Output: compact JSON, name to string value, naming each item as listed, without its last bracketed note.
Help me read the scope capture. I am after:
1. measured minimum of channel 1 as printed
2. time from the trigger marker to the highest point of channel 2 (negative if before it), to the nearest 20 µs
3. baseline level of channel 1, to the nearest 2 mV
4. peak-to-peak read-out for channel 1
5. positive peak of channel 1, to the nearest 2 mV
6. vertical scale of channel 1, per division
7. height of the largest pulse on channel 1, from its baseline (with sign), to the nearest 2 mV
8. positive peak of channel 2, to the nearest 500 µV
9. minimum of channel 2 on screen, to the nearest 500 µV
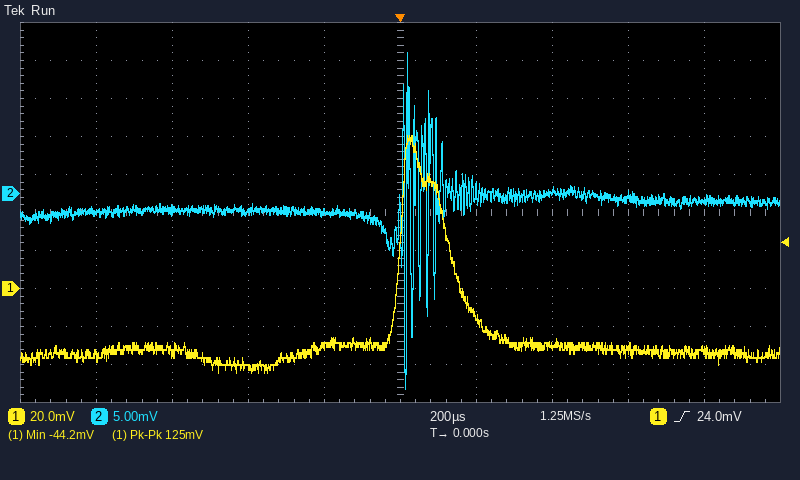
{"measured minimum of channel 1 as printed": "-44.2 mV", "time from the trigger marker to the highest point of channel 2 (negative if before it), to the nearest 20 µs": "+20 µs", "baseline level of channel 1, to the nearest 2 mV": "-32 mV", "peak-to-peak read-out for channel 1": "125 mV", "positive peak of channel 1, to the nearest 2 mV": "80 mV", "vertical scale of channel 1, per division": "20 mV", "height of the largest pulse on channel 1, from its baseline (with sign), to the nearest 2 mV": "+112 mV", "positive peak of channel 2, to the nearest 500 µV": "18.5 mV", "minimum of channel 2 on screen, to the nearest 500 µV": "-25.5 mV"}
